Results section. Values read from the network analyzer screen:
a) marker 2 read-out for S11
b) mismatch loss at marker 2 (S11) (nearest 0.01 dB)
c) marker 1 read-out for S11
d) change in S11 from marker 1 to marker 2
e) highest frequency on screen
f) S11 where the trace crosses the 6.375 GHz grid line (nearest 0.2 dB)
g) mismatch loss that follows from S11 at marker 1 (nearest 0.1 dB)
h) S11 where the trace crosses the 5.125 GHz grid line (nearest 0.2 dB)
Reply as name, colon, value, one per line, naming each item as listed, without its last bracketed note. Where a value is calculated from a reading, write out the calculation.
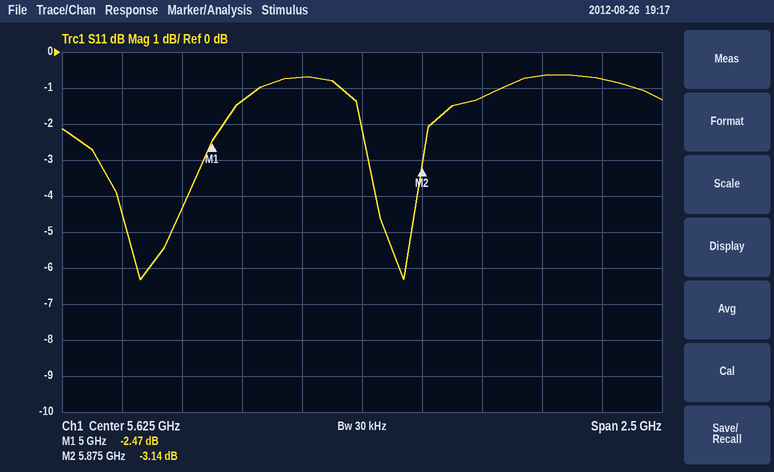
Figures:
marker 2 read-out for S11: -3.14 dB
mismatch loss at marker 2 (S11): −10 log10(1 − 10^(-3.14/10)) ≈ 2.88 dB
marker 1 read-out for S11: -2.47 dB
change in S11 from marker 1 to marker 2: -3.14 − (-2.47) = -0.67 dB
highest frequency on screen: 6.875 GHz
S11 where the trace crosses the 6.375 GHz grid line: -0.6 dB
mismatch loss that follows from S11 at marker 1: −10 log10(1 − 10^(-2.47/10)) ≈ 3.6 dB
S11 where the trace crosses the 5.125 GHz grid line: -1.4 dB
